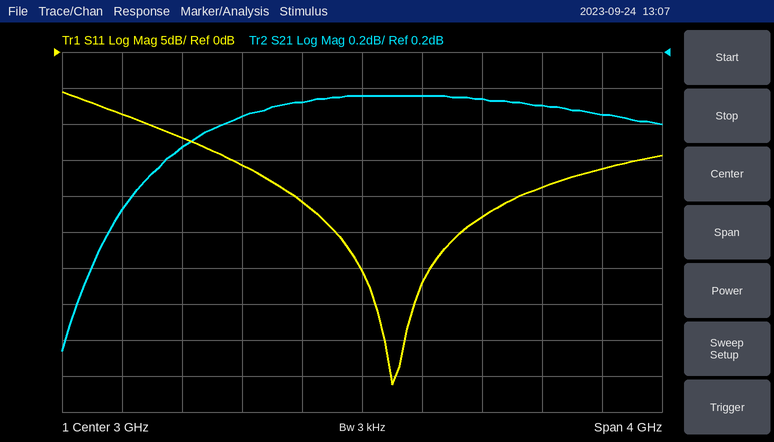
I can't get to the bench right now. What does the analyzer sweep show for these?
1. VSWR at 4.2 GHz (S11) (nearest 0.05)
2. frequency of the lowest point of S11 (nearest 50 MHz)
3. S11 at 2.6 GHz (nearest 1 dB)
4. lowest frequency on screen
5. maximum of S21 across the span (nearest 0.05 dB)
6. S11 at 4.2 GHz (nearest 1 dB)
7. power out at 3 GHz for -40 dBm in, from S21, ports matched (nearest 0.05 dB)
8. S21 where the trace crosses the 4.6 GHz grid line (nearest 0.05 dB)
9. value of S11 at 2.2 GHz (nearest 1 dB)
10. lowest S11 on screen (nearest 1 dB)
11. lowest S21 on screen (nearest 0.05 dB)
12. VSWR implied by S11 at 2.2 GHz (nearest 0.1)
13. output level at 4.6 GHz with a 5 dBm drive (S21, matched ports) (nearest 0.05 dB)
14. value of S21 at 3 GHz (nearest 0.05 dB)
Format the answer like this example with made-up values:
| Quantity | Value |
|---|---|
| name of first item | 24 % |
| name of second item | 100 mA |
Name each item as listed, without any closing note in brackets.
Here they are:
| Quantity | Value |
|---|---|
| VSWR at 4.2 GHz (S11) | 1.25 |
| frequency of the lowest point of S11 | 3.20 GHz |
| S11 at 2.6 GHz | -21 dB |
| lowest frequency on screen | 1 GHz |
| maximum of S21 across the span | -0.05 dB |
| S11 at 4.2 GHz | -19 dB |
| power out at 3 GHz for -40 dBm in, from S21, ports matched | -40.05 dBm |
| S21 where the trace crosses the 4.6 GHz grid line | -0.15 dB |
| value of S11 at 2.2 GHz | -16 dB |
| lowest S11 on screen | -46 dB |
| lowest S21 on screen | -1.45 dB |
| VSWR implied by S11 at 2.2 GHz | 1.4 |
| output level at 4.6 GHz with a 5 dBm drive (S21, matched ports) | 4.85 dBm |
| value of S21 at 3 GHz | -0.05 dB |
